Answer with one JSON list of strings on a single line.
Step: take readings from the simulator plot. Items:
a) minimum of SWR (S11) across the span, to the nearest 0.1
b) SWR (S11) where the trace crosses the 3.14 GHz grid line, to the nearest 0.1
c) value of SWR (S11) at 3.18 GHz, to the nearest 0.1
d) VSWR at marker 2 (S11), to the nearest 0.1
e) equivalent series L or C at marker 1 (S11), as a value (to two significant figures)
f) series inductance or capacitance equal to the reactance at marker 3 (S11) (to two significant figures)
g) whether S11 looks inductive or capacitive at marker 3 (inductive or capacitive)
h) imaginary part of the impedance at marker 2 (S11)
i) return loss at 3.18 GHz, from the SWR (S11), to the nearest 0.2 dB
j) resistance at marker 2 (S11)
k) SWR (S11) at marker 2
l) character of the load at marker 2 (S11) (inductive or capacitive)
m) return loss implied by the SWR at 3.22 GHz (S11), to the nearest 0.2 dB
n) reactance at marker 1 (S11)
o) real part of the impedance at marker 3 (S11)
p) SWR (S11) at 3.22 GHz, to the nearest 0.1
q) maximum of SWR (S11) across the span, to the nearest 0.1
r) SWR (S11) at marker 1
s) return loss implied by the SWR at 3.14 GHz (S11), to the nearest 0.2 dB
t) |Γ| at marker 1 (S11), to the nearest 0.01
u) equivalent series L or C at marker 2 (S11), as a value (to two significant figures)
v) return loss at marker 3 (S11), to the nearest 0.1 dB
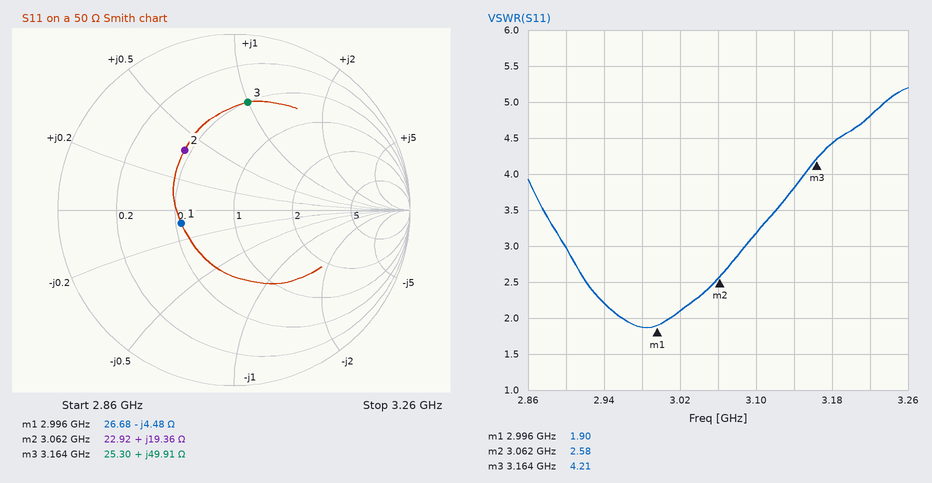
["1.9", "3.8", "4.4", "2.6", "12 pF", "2.5 nH", "inductive", "+19.36 Ω", "4.0 dB", "22.92 Ω", "2.58", "inductive", "3.6 dB", "-4.48 Ω", "25.30 Ω", "4.8", "5.2", "1.90", "4.6 dB", "0.31", "1.0 nH", "4.2 dB"]
